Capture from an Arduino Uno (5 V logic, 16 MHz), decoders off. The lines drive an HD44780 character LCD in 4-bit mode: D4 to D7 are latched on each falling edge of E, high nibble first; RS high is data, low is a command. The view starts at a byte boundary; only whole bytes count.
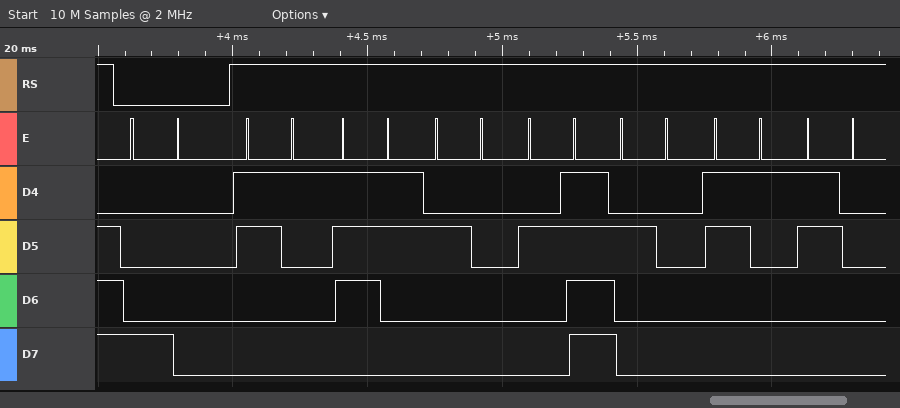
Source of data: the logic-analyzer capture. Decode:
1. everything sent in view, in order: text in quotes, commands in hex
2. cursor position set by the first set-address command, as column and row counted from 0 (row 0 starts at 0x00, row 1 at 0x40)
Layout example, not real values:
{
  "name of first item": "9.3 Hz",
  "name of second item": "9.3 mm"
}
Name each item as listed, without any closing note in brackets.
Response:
{
  "everything sent in view, in order: text in quotes, commands in hex": "0x80 \"1s / 10\"",
  "cursor position set by the first set-address command, as column and row counted from 0": "column 0, row 0"
}
